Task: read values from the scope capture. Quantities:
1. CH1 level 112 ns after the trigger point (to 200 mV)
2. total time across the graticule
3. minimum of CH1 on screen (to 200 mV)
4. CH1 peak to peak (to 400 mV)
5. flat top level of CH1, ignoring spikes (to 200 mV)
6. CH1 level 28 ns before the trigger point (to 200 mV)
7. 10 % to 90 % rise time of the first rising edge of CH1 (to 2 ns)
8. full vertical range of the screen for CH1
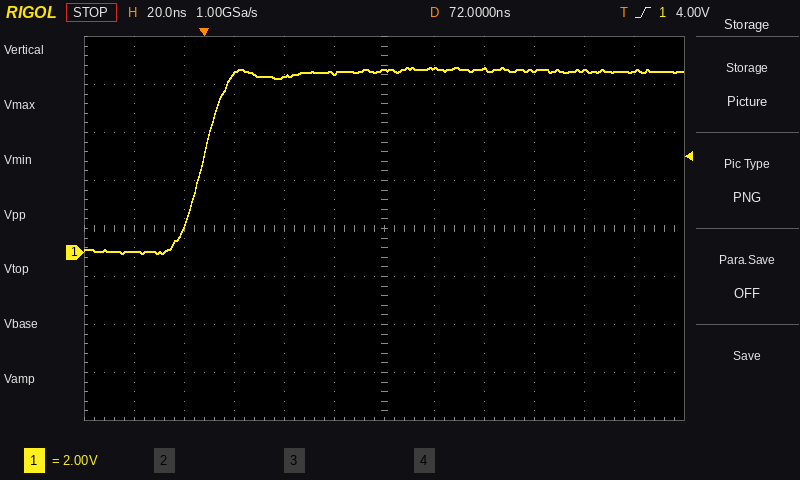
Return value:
7.6 V
240 ns
0.0 V
7.6 V
7.6 V
0.0 V
18 ns
16 V
